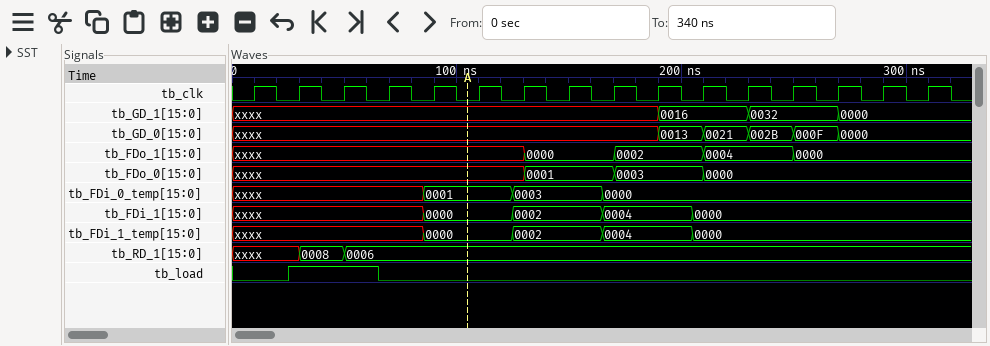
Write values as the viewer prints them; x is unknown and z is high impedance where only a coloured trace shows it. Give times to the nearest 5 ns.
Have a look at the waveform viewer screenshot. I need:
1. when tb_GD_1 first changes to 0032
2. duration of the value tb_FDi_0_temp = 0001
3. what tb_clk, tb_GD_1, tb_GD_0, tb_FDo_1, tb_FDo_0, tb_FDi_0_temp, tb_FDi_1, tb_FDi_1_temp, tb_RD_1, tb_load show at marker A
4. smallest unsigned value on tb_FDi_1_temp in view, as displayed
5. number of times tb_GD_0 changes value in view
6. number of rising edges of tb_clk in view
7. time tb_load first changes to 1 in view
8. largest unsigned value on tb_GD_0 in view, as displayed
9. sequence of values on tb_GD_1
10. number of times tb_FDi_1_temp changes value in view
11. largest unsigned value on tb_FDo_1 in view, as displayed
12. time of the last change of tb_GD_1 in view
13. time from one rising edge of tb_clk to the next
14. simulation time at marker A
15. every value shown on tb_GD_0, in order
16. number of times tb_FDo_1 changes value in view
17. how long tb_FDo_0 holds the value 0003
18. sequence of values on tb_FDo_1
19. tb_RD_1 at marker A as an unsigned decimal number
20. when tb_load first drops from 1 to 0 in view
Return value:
230 ns
40 ns
tb_clk=0, tb_GD_1=xxxx, tb_GD_0=xxxx, tb_FDo_1=xxxx, tb_FDo_0=xxxx, tb_FDi_0_temp=0001, tb_FDi_1=0000, tb_FDi_1_temp=0000, tb_RD_1=0006, tb_load=0
0000
5
16
25 ns
002B
xxxx, 0016, 0032, 0000
4
0004
270 ns
20 ns
105 ns
xxxx, 0013, 0021, 002B, 000F, 0000
4
40 ns
xxxx, 0000, 0002, 0004, 0000
6
65 ns
